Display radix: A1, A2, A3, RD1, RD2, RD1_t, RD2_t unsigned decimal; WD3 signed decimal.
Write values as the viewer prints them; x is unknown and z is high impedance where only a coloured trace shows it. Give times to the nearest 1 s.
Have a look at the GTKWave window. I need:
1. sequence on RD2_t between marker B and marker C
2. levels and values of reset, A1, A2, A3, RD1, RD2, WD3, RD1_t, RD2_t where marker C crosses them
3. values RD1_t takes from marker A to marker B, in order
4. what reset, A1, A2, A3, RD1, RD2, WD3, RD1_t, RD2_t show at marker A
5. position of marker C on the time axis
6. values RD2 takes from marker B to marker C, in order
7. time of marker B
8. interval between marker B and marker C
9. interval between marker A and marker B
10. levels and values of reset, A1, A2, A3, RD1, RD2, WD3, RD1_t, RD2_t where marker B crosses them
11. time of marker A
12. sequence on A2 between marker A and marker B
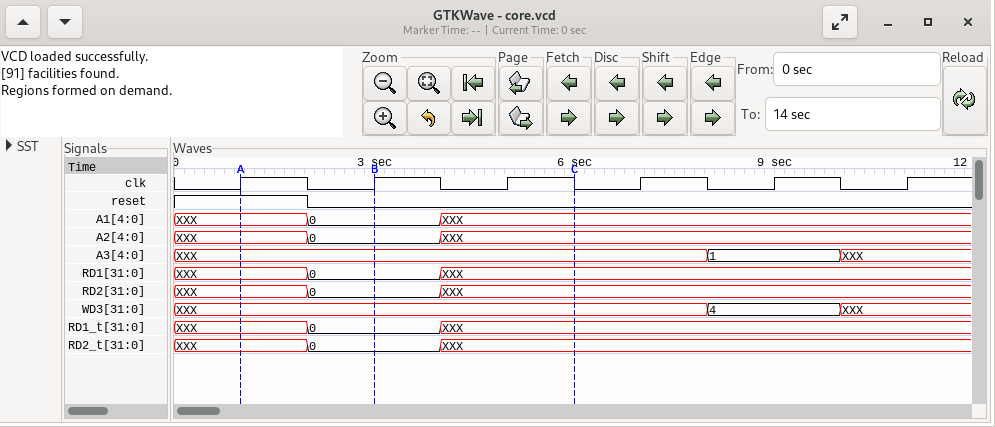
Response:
0, XXX
reset=0, A1=XXX, A2=XXX, A3=XXX, RD1=XXX, RD2=XXX, WD3=XXX, RD1_t=XXX, RD2_t=XXX
XXX, 0
reset=1, A1=XXX, A2=XXX, A3=XXX, RD1=XXX, RD2=XXX, WD3=XXX, RD1_t=XXX, RD2_t=XXX
6 s
0, XXX
3 s
3 s
2 s
reset=0, A1=0, A2=0, A3=XXX, RD1=0, RD2=0, WD3=XXX, RD1_t=0, RD2_t=0
1 s
XXX, 0
